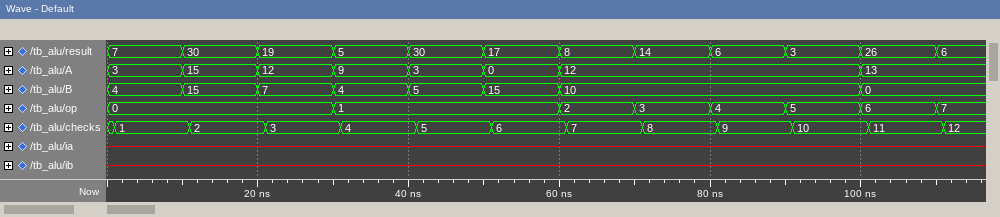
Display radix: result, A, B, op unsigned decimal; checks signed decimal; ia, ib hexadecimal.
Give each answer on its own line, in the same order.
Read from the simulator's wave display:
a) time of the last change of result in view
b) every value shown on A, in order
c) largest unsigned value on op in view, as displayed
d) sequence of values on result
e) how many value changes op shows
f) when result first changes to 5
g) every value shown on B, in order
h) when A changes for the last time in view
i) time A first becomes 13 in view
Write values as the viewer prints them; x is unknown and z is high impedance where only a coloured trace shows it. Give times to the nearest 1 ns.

110 ns
3, 15, 12, 9, 3, 0, 12, 13
7
7, 30, 19, 5, 30, 17, 8, 14, 6, 3, 26, 6
7
30 ns
4, 15, 7, 4, 5, 15, 10, 0
100 ns
100 ns
